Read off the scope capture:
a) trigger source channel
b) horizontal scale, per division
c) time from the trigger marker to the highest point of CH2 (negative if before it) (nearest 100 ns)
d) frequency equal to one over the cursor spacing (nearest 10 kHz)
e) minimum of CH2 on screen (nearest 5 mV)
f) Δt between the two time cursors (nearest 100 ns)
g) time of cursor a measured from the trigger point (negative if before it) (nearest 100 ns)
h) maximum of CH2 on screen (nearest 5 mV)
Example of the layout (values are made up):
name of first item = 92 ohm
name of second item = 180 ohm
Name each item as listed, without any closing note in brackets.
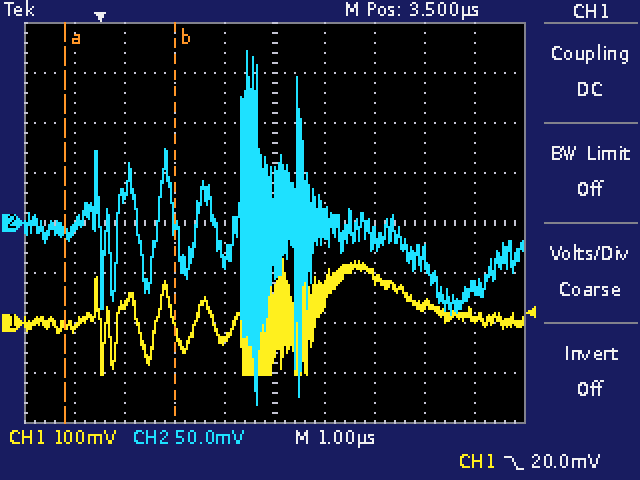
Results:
trigger source channel = CH1
horizontal scale, per division = 1 µs
time from the trigger marker to the highest point of CH2 (negative if before it) = +3.0 µs
frequency equal to one over the cursor spacing = 450 kHz
minimum of CH2 on screen = -180 mV
Δt between the two time cursors = 2.2 µs
time of cursor a measured from the trigger point (negative if before it) = -700 ns
maximum of CH2 on screen = 170 mV
